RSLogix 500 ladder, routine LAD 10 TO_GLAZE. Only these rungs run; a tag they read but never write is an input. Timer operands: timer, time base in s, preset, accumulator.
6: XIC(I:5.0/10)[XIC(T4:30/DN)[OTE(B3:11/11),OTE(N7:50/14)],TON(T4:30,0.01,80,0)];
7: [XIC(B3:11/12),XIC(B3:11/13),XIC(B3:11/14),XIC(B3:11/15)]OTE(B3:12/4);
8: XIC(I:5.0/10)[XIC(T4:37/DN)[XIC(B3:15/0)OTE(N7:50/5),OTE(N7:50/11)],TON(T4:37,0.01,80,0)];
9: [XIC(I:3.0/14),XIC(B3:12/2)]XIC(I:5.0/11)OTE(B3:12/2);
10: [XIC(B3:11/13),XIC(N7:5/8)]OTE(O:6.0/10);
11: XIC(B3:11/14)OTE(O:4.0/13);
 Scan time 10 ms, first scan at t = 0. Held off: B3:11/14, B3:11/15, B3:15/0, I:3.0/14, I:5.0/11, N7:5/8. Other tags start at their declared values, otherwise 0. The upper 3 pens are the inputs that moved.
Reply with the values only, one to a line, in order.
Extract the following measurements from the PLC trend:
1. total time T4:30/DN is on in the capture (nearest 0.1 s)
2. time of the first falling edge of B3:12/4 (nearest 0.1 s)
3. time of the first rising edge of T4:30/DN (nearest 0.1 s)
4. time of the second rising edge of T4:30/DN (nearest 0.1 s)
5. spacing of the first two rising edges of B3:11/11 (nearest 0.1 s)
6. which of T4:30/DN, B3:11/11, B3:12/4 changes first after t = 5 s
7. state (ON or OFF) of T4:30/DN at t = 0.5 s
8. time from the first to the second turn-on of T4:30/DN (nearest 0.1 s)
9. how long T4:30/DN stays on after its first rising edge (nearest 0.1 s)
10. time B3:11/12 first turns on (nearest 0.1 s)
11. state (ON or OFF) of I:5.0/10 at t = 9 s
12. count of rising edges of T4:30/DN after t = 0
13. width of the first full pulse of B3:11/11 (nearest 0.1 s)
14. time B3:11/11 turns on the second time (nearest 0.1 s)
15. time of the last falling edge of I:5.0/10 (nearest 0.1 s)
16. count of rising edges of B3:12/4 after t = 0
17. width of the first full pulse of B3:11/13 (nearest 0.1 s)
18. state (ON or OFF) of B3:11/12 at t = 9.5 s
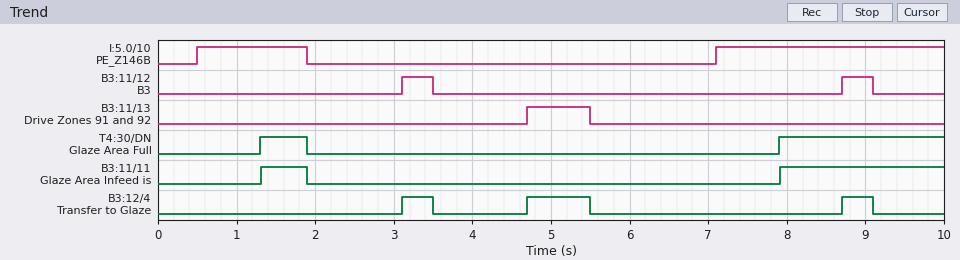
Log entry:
2.7 s
3.5 s
1.3 s
7.9 s
6.6 s
B3:12/4
OFF
6.6 s
0.6 s
3.1 s
ON
2
0.6 s
7.9 s
1.9 s
3
0.8 s
OFF
